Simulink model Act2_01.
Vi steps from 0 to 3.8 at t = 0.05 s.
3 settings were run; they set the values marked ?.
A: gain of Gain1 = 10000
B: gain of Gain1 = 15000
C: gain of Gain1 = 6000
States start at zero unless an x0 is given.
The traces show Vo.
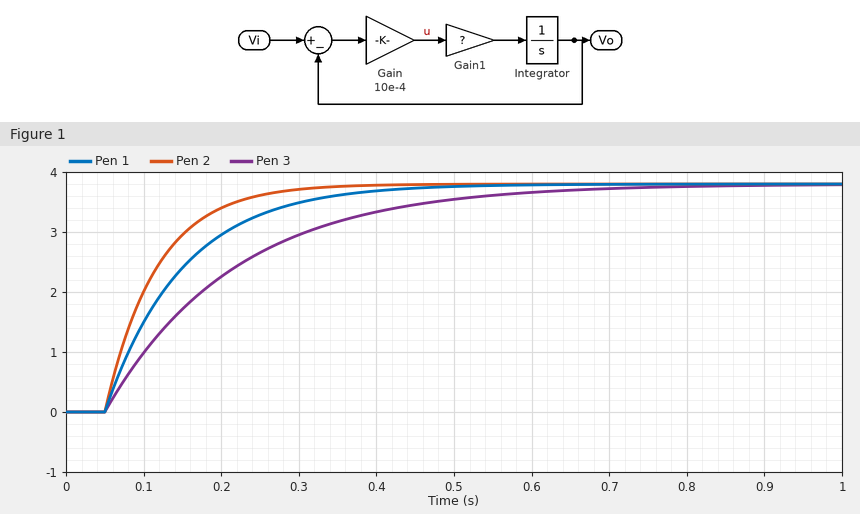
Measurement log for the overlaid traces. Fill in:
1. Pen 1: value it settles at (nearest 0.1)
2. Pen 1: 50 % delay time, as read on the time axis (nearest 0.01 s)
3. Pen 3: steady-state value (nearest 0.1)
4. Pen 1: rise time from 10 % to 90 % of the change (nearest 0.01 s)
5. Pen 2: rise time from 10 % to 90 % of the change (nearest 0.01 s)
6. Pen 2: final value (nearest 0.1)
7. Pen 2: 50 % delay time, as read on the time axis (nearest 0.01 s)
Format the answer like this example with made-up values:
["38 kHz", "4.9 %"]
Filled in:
["3.8", "0.12 s", "3.8", "0.22 s", "0.15 s", "3.8", "0.10 s"]
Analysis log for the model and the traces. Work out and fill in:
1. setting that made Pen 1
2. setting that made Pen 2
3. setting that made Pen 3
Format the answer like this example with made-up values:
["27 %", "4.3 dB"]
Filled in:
["A", "B", "C"]
